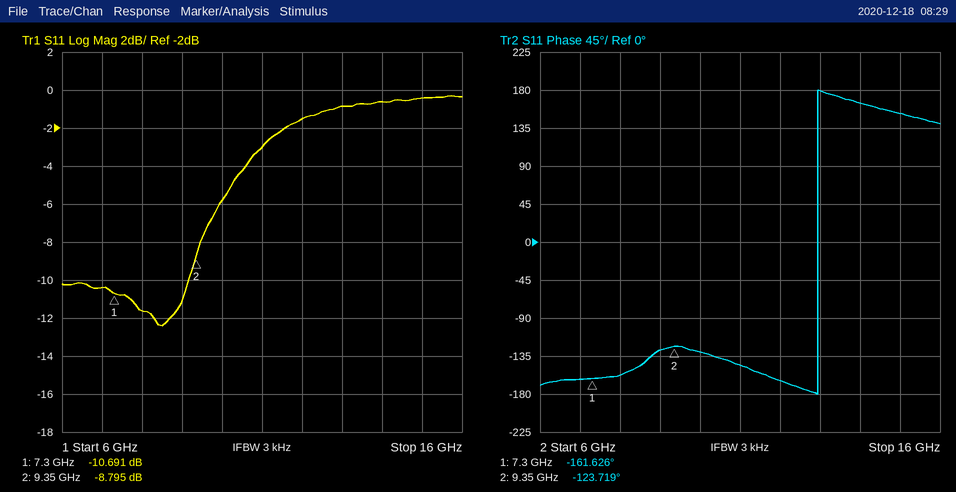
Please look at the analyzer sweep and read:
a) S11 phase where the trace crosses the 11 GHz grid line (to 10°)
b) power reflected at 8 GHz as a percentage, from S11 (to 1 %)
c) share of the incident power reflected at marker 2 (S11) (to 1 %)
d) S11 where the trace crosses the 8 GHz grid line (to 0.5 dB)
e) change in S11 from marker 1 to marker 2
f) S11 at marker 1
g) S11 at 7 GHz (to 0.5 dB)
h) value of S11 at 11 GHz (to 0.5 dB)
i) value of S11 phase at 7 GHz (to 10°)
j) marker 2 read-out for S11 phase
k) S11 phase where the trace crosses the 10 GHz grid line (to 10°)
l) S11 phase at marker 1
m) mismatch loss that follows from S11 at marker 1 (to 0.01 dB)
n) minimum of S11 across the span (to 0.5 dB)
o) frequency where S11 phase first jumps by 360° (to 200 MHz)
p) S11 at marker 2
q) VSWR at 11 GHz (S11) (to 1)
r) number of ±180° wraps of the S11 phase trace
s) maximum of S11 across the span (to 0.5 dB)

-150°
7 %
13 %
-11.5 dB
1.896 dB
-10.691 dB
-10.5 dB
-3.0 dB
-160°
-123.719°
-130°
-161.626°
0.39 dB
-12.5 dB
13.0 GHz
-8.795 dB
6
1
-0.5 dB
